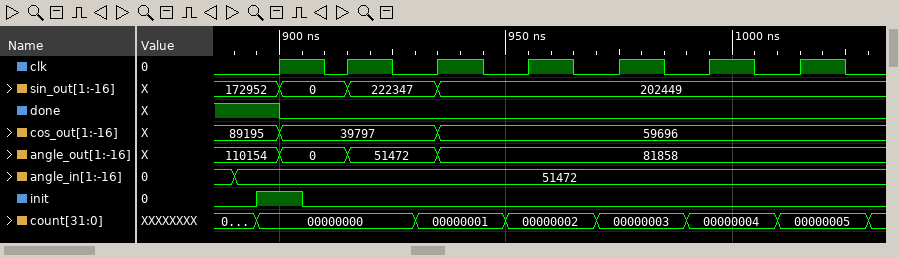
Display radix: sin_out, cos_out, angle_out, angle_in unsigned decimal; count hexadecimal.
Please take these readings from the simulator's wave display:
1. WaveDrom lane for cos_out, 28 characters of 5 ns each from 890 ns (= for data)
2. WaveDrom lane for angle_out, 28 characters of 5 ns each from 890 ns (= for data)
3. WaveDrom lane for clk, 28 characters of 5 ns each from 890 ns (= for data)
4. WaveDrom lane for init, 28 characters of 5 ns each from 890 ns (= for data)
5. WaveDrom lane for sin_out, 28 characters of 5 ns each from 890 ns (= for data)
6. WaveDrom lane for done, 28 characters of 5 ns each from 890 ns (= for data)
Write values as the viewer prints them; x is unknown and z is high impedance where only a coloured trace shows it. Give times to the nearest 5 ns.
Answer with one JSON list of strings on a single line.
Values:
["{name: 'cos_out', wave: '=.=......=..................', data: '89195 39797 59696'}", "{name: 'angle_out', wave: '=.=..=...=..................', data: '110154 0 51472 81858'}", "{name: 'clk', wave: '0.1.01.0.1.0.1.0.1.0.1.0.1.0'}", "{name: 'init', wave: '01.0........................'}", "{name: 'sin_out', wave: '=.=..=...=..................', data: '172952 0 222347 202449'}", "{name: 'done', wave: '1.0.........................'}"]
